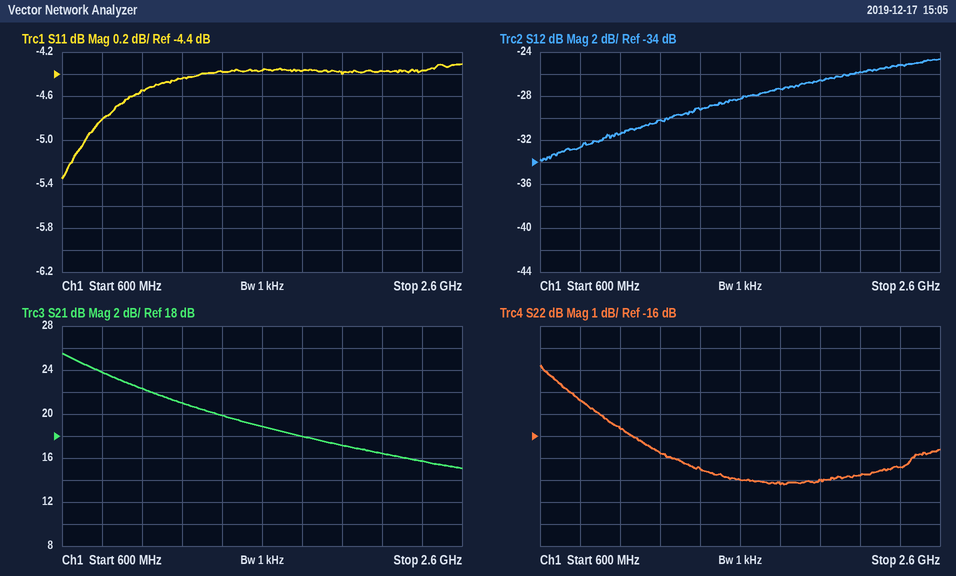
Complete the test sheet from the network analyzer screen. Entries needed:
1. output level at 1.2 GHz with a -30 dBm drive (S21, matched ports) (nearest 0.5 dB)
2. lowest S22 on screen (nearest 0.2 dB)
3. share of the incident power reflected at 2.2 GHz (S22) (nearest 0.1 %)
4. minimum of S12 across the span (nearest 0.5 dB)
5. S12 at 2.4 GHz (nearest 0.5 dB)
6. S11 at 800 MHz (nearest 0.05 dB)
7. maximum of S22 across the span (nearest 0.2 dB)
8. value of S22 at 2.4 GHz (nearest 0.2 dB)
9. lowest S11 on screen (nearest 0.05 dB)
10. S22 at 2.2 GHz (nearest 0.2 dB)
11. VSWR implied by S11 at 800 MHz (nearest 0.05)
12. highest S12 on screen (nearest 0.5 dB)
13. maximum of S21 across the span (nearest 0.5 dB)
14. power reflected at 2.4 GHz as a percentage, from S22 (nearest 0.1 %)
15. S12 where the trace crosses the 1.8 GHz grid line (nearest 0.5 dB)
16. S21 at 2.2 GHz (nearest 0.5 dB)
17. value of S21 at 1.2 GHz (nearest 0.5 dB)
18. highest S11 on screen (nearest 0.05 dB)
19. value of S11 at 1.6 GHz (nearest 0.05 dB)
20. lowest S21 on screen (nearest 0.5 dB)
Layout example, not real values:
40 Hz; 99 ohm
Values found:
-9.0 dBm; -18.2 dB; 1.7 %; -34.0 dB; -25.0 dB; -4.80 dB; -12.8 dB; -17.4 dB; -5.35 dB; -17.8 dB; 3.70; -24.5 dB; 25.5 dB; 1.8 %; -27.5 dB; 16.5 dB; 21.0 dB; -4.30 dB; -4.35 dB; 15.0 dB
